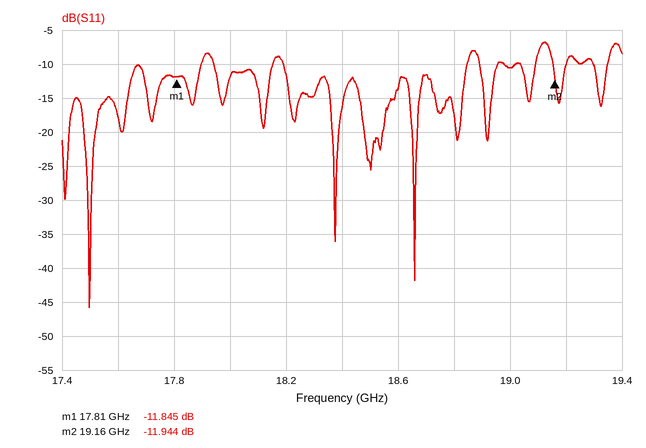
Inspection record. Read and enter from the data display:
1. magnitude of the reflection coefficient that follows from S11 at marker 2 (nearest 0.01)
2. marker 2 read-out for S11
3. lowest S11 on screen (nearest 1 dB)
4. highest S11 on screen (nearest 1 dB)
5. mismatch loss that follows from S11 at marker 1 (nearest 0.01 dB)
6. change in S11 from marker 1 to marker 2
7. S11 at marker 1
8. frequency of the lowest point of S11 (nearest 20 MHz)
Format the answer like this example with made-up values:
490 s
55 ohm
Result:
0.25
-11.944 dB
-46 dB
-7 dB
0.29 dB
-0.099 dB
-11.845 dB
17.50 GHz
